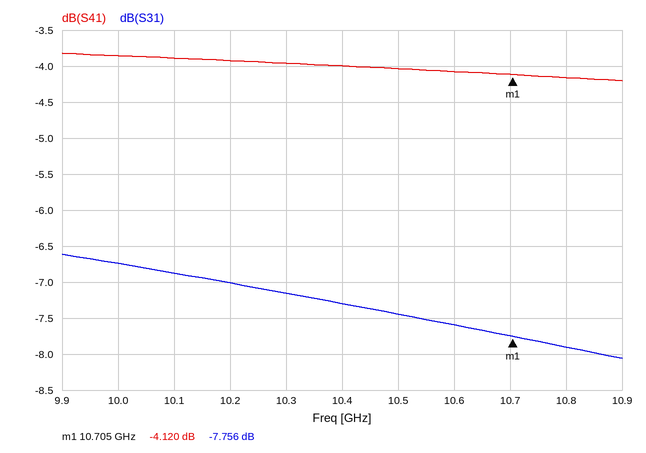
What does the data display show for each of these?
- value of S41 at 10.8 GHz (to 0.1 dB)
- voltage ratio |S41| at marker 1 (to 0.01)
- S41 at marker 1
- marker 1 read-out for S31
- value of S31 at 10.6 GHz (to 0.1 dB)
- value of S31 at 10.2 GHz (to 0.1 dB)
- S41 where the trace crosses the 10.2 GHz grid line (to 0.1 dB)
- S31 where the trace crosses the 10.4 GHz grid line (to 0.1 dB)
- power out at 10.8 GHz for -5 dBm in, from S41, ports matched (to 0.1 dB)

-4.2 dB
0.62
-4.120 dB
-7.756 dB
-7.6 dB
-7.0 dB
-3.9 dB
-7.3 dB
-9.2 dBm
